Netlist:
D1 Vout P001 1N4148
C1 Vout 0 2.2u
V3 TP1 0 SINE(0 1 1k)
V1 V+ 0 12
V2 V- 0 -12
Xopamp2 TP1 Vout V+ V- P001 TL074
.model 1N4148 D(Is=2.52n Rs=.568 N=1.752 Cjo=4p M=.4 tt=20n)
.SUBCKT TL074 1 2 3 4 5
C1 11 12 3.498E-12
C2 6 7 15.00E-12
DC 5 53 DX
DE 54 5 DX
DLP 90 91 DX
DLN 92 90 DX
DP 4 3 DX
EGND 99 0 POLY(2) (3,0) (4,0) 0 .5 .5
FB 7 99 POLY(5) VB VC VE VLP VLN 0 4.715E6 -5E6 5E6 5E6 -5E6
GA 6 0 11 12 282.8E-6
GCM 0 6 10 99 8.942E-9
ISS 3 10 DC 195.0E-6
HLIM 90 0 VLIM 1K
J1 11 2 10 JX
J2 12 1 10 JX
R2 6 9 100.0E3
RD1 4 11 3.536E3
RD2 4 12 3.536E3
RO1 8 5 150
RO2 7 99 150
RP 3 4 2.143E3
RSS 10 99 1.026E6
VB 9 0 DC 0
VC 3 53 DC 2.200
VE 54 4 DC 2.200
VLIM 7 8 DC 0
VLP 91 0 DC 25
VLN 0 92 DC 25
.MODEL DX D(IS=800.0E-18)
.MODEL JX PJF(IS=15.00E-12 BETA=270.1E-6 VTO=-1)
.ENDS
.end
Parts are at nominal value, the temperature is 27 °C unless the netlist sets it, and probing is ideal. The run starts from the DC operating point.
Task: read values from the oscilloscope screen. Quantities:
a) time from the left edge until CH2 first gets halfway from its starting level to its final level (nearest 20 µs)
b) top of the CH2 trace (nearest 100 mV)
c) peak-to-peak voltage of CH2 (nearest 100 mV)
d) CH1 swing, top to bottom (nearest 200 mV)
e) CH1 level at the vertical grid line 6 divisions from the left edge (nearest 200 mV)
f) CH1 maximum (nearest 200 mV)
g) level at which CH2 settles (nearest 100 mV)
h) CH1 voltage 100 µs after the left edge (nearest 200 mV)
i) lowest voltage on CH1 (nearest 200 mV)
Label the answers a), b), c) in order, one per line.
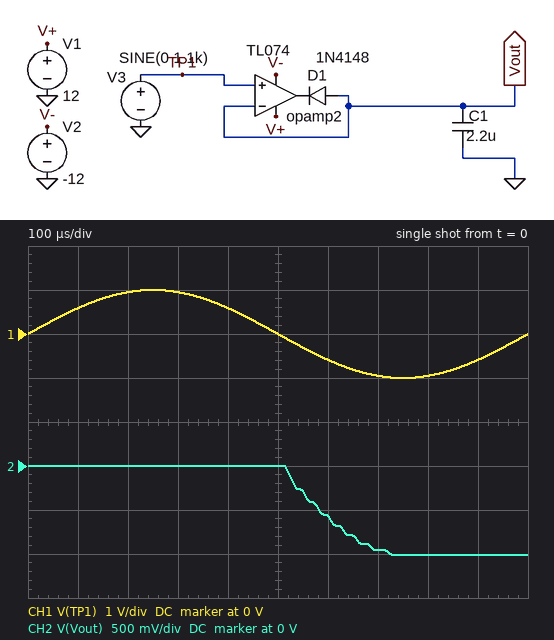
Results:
a) 580 µs
b) 0 V
c) 1.0 V
d) 2.0 V
e) -600 mV
f) 1.0 V
g) -1.0 V
h) 600 mV
i) -1.0 V
